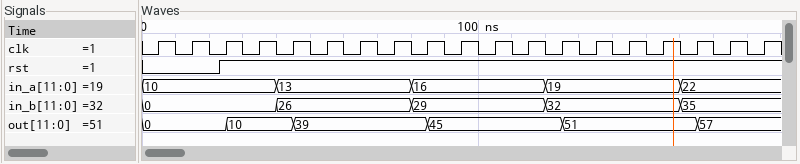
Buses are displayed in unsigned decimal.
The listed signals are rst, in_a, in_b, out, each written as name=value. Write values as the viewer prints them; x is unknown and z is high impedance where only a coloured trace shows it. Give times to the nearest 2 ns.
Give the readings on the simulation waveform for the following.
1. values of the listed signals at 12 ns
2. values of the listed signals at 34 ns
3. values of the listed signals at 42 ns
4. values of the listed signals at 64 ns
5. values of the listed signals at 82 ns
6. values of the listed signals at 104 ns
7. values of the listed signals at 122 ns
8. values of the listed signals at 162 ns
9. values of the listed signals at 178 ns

rst=0, in_a=10, in_b=0, out=0
rst=1, in_a=10, in_b=0, out=10
rst=1, in_a=13, in_b=26, out=10
rst=1, in_a=13, in_b=26, out=39
rst=1, in_a=16, in_b=29, out=39
rst=1, in_a=16, in_b=29, out=45
rst=1, in_a=19, in_b=32, out=45
rst=1, in_a=22, in_b=35, out=51
rst=1, in_a=22, in_b=35, out=57
